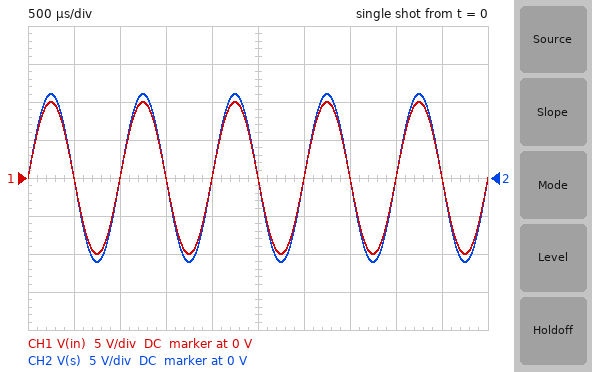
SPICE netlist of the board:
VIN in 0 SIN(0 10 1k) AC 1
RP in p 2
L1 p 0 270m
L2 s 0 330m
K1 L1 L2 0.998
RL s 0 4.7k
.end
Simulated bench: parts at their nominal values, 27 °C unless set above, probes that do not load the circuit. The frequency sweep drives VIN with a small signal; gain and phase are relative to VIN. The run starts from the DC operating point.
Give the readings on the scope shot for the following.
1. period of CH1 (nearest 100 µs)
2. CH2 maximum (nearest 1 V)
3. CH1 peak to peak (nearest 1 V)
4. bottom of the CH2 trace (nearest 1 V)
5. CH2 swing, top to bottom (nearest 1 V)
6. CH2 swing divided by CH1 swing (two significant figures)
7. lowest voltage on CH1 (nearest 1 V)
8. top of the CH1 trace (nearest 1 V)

1.0 ms
11 V
20 V
-11 V
22 V
1.1
-10 V
10 V
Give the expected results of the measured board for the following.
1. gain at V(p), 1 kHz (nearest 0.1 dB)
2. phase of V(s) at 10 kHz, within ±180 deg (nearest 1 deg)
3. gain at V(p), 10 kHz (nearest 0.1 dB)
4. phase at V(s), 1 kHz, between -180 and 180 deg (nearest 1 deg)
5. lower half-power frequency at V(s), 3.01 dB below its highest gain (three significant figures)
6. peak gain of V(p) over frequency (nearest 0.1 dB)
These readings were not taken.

0 dB
-1 deg
0 dB
0 deg
1.18 Hz
0 dB
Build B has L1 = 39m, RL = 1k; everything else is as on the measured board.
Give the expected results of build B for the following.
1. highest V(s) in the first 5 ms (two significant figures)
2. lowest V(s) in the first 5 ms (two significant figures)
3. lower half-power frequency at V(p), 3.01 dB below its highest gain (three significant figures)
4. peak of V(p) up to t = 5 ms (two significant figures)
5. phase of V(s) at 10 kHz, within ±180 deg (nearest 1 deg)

28 V
-29 V
8.30 Hz
9.8 V
-5 deg
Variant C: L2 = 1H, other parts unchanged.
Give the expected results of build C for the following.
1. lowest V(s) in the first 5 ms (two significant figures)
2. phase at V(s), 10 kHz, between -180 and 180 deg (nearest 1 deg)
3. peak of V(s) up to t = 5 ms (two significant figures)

-19 V
-3 deg
19 V
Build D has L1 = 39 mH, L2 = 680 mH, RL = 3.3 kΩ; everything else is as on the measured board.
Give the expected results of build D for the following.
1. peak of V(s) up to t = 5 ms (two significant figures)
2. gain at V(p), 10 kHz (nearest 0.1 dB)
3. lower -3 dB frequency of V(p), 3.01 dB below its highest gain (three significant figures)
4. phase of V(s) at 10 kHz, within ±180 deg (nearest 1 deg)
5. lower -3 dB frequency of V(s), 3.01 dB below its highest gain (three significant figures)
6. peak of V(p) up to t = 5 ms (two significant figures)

41 V
-0.1 dB
8.25 Hz
-3 deg
8.08 Hz
9.8 V
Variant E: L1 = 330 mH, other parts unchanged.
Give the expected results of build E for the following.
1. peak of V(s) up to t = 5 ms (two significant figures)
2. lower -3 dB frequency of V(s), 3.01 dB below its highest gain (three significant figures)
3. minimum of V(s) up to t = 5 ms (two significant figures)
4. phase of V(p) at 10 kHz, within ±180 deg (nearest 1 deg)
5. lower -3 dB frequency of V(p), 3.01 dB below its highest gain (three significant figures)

10 V
964 mHz
-10 V
0 deg
965 mHz
